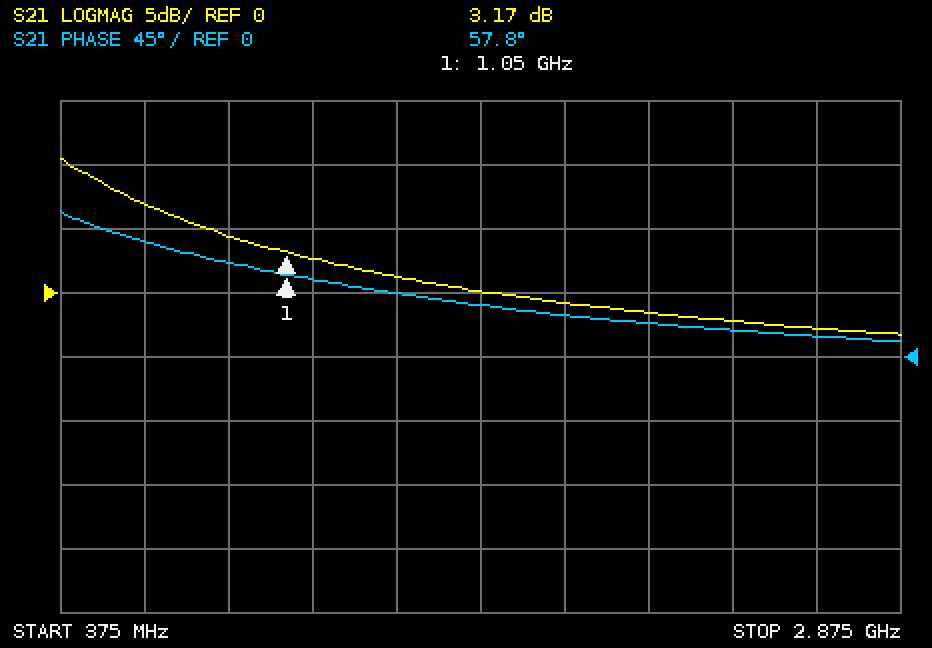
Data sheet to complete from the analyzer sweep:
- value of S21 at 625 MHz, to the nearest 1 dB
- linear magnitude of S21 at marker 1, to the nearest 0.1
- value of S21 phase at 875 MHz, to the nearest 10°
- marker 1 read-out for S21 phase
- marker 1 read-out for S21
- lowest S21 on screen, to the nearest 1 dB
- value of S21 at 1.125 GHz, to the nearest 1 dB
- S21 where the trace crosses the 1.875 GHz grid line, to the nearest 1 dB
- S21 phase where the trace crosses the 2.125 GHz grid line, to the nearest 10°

7 dB
1.4
70°
57.8°
3.17 dB
-3 dB
3 dB
-1 dB
20°
